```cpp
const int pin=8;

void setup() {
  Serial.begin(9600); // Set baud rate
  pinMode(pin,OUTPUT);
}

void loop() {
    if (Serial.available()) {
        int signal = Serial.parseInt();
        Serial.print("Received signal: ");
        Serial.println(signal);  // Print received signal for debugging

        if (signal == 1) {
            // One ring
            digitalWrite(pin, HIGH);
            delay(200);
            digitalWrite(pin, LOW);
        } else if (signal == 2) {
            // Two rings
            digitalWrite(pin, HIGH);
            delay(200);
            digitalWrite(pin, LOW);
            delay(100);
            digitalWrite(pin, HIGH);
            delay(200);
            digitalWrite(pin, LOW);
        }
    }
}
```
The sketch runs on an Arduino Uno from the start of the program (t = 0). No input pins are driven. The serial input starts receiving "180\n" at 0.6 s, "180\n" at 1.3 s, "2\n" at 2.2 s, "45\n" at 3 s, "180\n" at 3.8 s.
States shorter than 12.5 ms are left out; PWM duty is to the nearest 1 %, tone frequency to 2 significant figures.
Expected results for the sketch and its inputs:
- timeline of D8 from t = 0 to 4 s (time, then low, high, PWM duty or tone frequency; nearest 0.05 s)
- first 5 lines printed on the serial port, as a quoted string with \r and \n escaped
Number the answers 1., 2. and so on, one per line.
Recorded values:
1. 0 s low; 2.2 s high; 2.4 s low; 2.5 s high; 2.7 s low
2. "Received signal: 180\r\nReceived signal: 180\r\nReceived signal: 2\r\nReceived signal: 45\r\nReceived signal: 180\r\n"
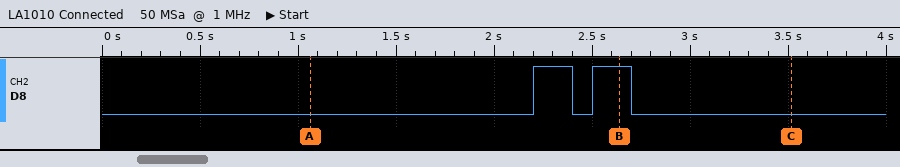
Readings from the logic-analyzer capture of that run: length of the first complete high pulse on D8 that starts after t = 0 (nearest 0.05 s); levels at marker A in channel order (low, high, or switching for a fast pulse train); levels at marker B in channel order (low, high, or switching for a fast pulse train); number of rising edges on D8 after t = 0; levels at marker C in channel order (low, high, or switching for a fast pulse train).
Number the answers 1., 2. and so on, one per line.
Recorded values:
1. 0.20 s
2. D8 low
3. D8 high
4. 2
5. D8 low
